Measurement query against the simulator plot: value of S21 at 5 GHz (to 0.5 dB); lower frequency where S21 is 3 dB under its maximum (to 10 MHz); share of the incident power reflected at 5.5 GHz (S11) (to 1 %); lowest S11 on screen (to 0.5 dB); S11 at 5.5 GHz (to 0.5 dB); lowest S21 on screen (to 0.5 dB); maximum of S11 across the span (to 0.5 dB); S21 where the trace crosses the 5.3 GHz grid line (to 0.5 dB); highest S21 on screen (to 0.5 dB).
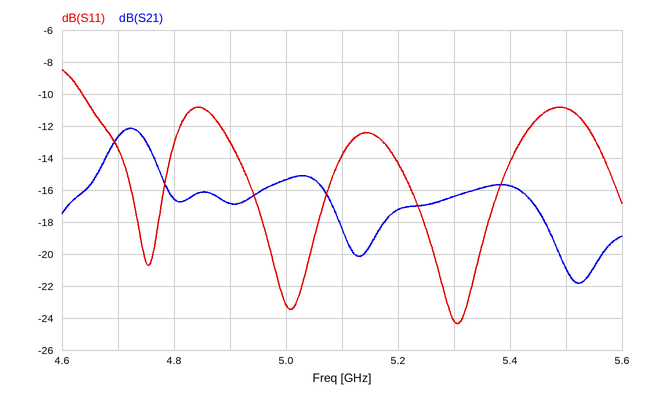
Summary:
-15.5 dB
4.66 GHz
8 %
-24.5 dB
-11.0 dB
-22.0 dB
-8.5 dB
-16.5 dB
-12.0 dB
